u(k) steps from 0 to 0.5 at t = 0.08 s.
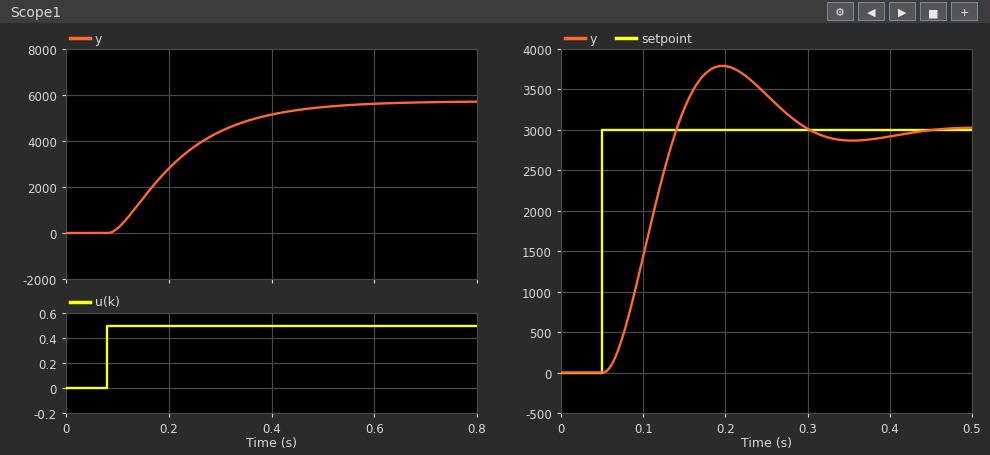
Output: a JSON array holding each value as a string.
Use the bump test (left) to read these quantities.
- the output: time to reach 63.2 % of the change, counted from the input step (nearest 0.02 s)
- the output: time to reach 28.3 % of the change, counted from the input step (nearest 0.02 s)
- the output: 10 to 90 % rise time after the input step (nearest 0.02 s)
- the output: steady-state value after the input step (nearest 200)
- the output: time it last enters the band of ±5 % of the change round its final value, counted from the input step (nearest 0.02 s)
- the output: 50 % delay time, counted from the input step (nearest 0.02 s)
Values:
["0.16 s", "0.08 s", "0.28 s", "5800", "0.40 s", "0.12 s"]
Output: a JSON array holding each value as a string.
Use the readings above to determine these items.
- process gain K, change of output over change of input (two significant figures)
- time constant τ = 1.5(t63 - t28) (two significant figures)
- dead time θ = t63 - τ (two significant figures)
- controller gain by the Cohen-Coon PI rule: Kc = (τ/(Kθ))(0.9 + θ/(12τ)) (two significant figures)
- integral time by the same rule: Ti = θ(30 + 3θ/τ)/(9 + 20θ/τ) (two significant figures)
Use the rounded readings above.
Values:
["12000", "0.12 s", "0.040 s", "0.00023", "0.079 s"]
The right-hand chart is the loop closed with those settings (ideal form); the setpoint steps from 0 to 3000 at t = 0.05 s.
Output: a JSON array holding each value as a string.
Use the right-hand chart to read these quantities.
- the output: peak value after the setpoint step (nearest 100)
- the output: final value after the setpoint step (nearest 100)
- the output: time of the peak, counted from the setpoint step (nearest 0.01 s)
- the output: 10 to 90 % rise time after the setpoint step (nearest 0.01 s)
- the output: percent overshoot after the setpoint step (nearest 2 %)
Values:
["3800", "3000", "0.15 s", "0.06 s", "26 %"]
